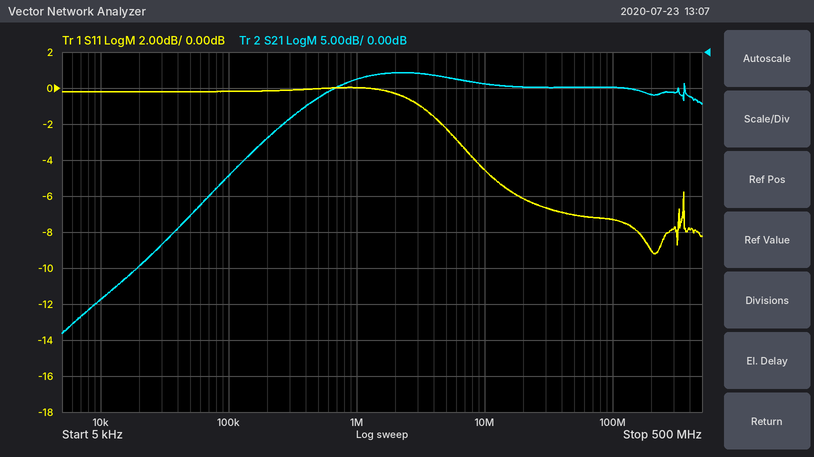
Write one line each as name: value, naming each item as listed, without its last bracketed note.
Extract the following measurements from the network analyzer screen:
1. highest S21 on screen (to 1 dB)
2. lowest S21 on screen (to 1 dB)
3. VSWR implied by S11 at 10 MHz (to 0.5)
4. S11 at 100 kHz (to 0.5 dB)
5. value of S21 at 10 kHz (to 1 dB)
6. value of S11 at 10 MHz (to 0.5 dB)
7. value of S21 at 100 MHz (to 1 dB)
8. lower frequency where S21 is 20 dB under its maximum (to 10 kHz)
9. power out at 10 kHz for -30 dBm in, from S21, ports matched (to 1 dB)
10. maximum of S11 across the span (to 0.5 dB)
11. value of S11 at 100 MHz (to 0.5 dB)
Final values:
highest S21 on screen: -3 dB
lowest S21 on screen: -39 dB
VSWR implied by S11 at 10 MHz: 4.0
S11 at 100 kHz: 0.0 dB
value of S21 at 10 kHz: -34 dB
value of S11 at 10 MHz: -4.5 dB
value of S21 at 100 MHz: -5 dB
lower frequency where S21 is 20 dB under its maximum: 50 kHz
power out at 10 kHz for -30 dBm in, from S21, ports matched: -64 dBm
maximum of S11 across the span: 0.0 dB
value of S11 at 100 MHz: -7.5 dB
